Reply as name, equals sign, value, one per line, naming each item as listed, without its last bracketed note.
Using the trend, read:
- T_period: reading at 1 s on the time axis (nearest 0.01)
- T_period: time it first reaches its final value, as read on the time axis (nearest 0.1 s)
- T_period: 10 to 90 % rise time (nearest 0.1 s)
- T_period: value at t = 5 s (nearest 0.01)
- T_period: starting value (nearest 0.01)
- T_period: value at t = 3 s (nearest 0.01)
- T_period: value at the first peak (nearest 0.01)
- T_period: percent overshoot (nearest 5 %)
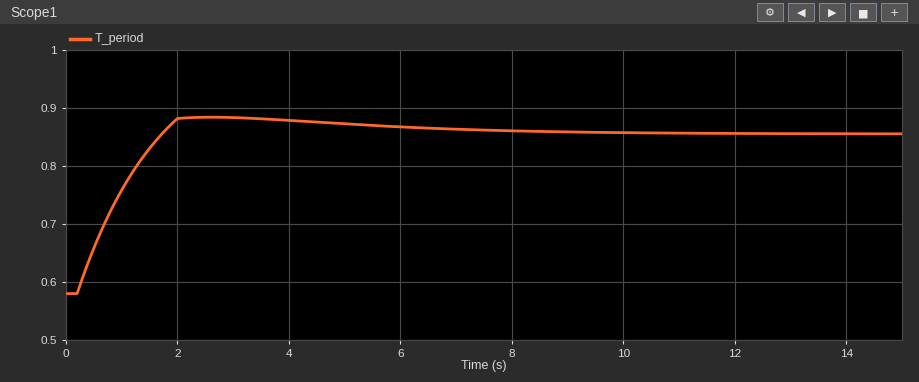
T_period: reading at 1 s on the time axis = 0.76
T_period: time it first reaches its final value, as read on the time axis = 1.7 s
T_period: 10 to 90 % rise time = 1.2 s
T_period: value at t = 5 s = 0.87
T_period: starting value = 0.58
T_period: value at t = 3 s = 0.88
T_period: value at the first peak = 0.88
T_period: percent overshoot = 10 %
